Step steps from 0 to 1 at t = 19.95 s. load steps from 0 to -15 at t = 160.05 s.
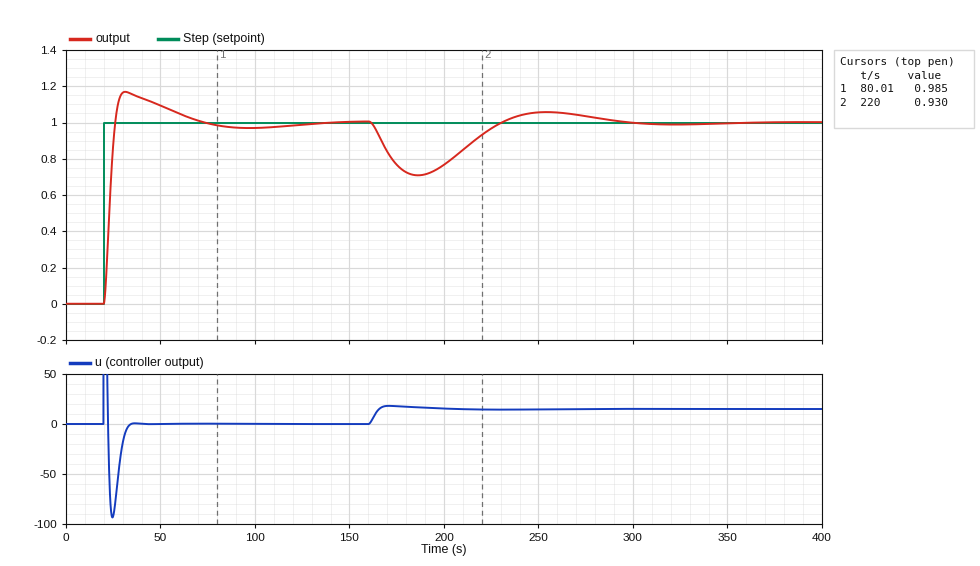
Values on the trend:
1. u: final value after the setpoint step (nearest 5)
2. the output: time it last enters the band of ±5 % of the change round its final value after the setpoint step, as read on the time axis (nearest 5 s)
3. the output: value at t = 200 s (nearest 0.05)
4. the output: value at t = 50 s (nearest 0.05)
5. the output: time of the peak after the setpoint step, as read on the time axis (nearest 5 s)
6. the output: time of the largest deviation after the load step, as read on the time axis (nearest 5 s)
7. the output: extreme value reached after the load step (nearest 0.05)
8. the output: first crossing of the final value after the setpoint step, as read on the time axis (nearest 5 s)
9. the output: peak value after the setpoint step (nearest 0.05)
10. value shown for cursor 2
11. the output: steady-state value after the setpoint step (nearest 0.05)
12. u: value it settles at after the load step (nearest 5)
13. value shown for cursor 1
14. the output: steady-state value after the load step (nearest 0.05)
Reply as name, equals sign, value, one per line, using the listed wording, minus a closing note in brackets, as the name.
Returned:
u: final value after the setpoint step = 0
the output: time it last enters the band of ±5 % of the change round its final value after the setpoint step, as read on the time axis = 60 s
the output: value at t = 200 s = 0.75
the output: value at t = 50 s = 1.10
the output: time of the peak after the setpoint step, as read on the time axis = 30 s
the output: time of the largest deviation after the load step, as read on the time axis = 185 s
the output: extreme value reached after the load step = 0.70
the output: first crossing of the final value after the setpoint step, as read on the time axis = 25 s
the output: peak value after the setpoint step = 1.15
value shown for cursor 2 = 0.930
the output: steady-state value after the setpoint step = 1.00
u: value it settles at after the load step = 15
value shown for cursor 1 = 0.985
the output: steady-state value after the load step = 1.00
